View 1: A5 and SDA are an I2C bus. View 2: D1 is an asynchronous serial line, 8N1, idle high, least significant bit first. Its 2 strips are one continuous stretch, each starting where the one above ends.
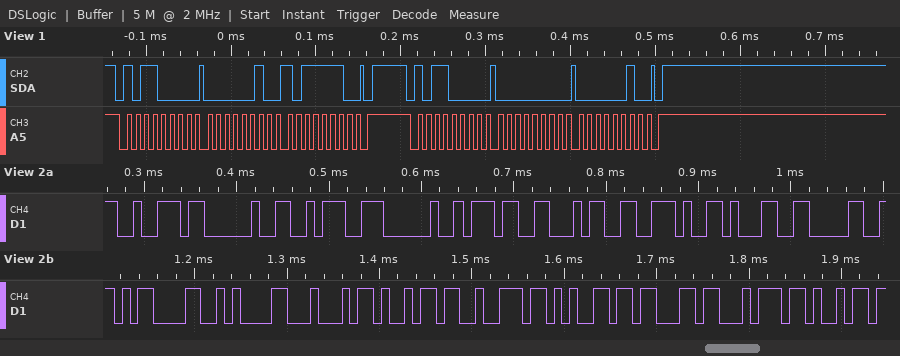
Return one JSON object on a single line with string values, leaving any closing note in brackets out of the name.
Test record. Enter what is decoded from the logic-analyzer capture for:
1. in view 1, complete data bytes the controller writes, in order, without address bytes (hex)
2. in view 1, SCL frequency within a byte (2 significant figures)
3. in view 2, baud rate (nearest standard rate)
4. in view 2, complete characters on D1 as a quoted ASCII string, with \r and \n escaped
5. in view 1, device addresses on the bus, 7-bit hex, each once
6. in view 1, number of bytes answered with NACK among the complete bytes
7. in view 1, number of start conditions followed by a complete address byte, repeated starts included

{"in view 1, complete data bytes the controller writes, in order, without address bytes": "02 BE 00 02", "in view 1, SCL frequency within a byte": "100 kHz", "in view 2, baud rate": "115200 baud", "in view 2, complete characters on D1 as a quoted ASCII string, with \\r and \\n escaped": "\"r : 74.10\\r\\nDirecti\"", "in view 1, device addresses on the bus, 7-bit hex, each once": "0x58", "in view 1, number of bytes answered with NACK among the complete bytes": "0", "in view 1, number of start conditions followed by a complete address byte, repeated starts included": "2"}
